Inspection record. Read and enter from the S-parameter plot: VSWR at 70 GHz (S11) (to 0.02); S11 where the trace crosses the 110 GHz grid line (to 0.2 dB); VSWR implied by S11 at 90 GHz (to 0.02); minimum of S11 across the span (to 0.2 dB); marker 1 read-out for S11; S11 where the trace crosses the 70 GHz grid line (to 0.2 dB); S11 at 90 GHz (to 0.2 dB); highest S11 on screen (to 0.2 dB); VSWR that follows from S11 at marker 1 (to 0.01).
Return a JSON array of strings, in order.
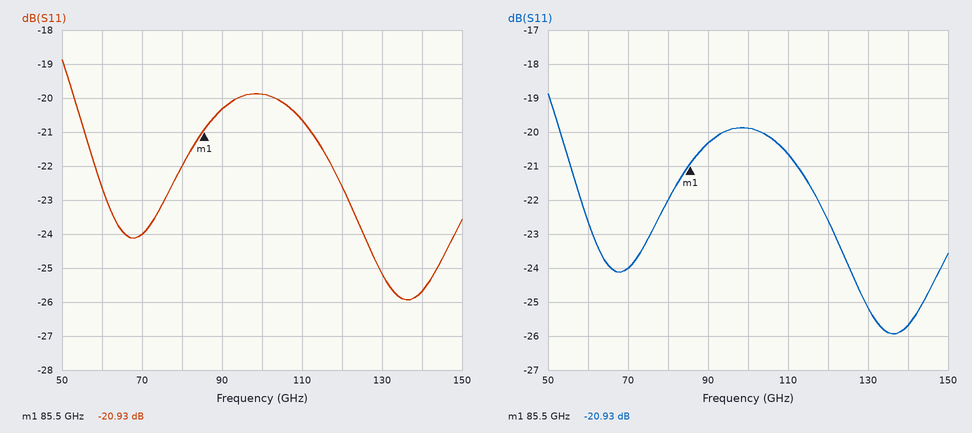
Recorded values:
["1.14", "-20.6 dB", "1.22", "-26.0 dB", "-20.93 dB", "-24.0 dB", "-20.4 dB", "-18.8 dB", "1.20"]
